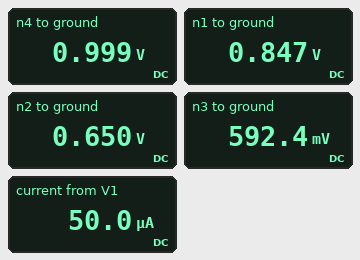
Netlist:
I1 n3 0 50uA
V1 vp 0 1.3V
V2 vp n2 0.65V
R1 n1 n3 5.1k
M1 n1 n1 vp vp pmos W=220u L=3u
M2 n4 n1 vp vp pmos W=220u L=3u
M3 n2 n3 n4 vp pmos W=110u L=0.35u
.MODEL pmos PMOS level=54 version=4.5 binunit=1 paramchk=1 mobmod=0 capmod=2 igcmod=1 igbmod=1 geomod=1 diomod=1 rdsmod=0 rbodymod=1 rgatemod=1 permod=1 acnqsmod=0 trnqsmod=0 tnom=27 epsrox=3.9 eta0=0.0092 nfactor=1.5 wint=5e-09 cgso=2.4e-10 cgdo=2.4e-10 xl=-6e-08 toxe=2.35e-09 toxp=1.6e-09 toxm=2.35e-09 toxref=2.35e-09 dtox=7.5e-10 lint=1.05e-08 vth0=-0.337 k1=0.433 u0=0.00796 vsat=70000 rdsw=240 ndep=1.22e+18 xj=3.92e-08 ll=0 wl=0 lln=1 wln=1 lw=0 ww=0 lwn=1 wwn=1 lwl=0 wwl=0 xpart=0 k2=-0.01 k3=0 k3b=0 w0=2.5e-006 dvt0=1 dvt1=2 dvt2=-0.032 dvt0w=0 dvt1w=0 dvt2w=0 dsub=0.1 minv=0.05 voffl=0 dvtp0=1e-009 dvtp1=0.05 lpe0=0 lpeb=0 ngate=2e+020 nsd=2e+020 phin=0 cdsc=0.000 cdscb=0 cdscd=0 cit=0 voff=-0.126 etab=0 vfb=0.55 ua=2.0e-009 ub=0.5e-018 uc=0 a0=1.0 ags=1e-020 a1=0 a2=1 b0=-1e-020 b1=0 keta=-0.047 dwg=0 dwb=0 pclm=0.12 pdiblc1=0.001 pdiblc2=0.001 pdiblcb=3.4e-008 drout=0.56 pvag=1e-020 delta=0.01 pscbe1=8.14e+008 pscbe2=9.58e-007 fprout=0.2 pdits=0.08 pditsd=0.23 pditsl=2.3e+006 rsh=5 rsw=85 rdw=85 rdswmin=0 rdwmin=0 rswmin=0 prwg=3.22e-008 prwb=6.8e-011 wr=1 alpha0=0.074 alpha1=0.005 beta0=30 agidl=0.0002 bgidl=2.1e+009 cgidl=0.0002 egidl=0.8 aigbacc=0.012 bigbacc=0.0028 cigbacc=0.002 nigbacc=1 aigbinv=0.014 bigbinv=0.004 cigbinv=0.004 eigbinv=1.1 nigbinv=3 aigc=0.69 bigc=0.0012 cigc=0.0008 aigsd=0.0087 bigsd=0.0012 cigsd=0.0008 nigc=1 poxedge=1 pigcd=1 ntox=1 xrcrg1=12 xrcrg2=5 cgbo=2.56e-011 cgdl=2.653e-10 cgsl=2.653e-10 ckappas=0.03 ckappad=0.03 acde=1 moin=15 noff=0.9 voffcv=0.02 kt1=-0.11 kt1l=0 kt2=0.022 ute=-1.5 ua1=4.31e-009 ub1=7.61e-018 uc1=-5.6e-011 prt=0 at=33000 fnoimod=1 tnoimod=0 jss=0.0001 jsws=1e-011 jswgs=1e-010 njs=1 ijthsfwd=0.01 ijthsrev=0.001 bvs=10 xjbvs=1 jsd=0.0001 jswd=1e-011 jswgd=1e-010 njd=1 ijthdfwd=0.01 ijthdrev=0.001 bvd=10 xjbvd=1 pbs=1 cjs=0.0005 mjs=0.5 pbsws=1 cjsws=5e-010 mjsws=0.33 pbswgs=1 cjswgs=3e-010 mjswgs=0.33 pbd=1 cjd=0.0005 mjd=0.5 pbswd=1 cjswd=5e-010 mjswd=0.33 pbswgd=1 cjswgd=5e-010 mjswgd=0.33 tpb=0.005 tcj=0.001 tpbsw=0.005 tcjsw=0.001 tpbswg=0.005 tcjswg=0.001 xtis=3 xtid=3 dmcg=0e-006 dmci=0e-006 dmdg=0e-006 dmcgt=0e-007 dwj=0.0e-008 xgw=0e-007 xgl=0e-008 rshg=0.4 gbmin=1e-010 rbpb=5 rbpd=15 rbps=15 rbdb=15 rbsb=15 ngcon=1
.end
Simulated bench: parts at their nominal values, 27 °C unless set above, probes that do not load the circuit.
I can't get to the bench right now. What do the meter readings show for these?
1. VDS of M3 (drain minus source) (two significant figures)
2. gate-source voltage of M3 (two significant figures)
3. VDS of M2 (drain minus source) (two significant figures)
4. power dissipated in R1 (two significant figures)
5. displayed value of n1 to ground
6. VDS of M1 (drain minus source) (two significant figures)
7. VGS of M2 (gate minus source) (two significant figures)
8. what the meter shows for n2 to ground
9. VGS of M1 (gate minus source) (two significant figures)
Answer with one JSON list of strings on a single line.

["-350 mV", "-410 mV", "-300 mV", "13 µW", "0.847 V", "-450 mV", "-450 mV", "0.650 V", "-450 mV"]
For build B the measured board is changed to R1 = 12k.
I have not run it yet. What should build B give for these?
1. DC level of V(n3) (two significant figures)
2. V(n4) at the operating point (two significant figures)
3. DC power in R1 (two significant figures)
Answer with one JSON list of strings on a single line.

["250 mV", "720 mV", "30 µW"]
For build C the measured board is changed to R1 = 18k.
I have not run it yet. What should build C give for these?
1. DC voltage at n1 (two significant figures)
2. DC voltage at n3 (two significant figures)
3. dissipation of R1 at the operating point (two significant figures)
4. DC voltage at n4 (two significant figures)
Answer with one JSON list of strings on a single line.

["850 mV", "-53 mV", "45 µW", "660 mV"]
